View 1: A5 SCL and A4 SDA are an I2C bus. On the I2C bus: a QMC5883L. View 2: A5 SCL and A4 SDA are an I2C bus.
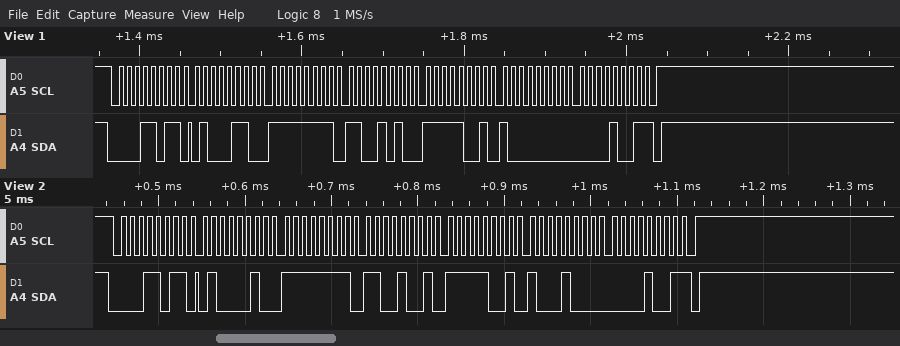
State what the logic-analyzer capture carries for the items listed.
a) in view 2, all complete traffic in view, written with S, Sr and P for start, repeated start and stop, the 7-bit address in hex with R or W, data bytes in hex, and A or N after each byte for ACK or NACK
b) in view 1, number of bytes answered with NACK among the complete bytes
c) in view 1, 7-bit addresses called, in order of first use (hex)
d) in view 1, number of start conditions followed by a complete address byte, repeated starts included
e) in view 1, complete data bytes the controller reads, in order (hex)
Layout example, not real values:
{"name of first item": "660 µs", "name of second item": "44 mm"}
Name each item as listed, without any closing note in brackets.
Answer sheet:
{"in view 2, all complete traffic in view, written with S, Sr and P for start, repeated start and stop, the 7-bit address in hex with R or W, data bytes in hex, and A or N after each byte for ACK or NACK": "S 0DR A 42 A FF A C9 A F9 A 88 A 09 N P", "in view 1, number of bytes answered with NACK among the complete bytes": "1", "in view 1, 7-bit addresses called, in order of first use": "0x0D", "in view 1, number of start conditions followed by a complete address byte, repeated starts included": "1", "in view 1, complete data bytes the controller reads, in order": "46 FF CA F9 80 09"}
